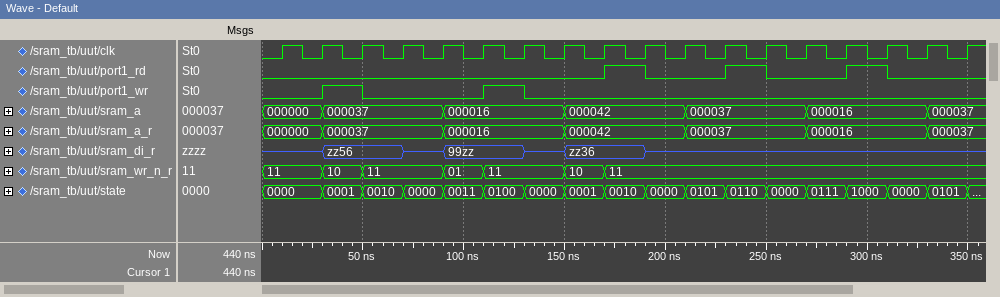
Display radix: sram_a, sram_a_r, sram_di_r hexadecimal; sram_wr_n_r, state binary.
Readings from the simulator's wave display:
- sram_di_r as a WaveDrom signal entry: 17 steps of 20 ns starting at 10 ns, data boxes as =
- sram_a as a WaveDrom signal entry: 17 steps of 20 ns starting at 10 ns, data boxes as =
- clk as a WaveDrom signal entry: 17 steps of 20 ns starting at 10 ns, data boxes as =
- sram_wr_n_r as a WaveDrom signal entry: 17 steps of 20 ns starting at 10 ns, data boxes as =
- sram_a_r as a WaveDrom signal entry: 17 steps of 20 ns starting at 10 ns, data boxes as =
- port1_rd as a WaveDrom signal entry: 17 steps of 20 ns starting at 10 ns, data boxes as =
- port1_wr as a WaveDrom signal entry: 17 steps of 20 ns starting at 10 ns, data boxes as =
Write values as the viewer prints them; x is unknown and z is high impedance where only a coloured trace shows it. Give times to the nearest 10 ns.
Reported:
{name: 'sram_di_r', wave: 'z=.z=.z=.z.......', data: 'zz56 99zz zz36'}
{name: 'sram_a', wave: '==..=..=..=..=..=', data: '000000 000037 000016 000042 000037 000016 000037'}
{name: 'clk', wave: 'p................'}
{name: 'sram_wr_n_r', wave: '===.==.==........', data: '11 10 11 01 11 10 11'}
{name: 'sram_a_r', wave: '==..=..=..=..=..=', data: '000000 000037 000016 000042 000037 000016 000037'}
{name: 'port1_rd', wave: '0.......10.10.10.'}
{name: 'port1_wr', wave: '010..10..........'}
